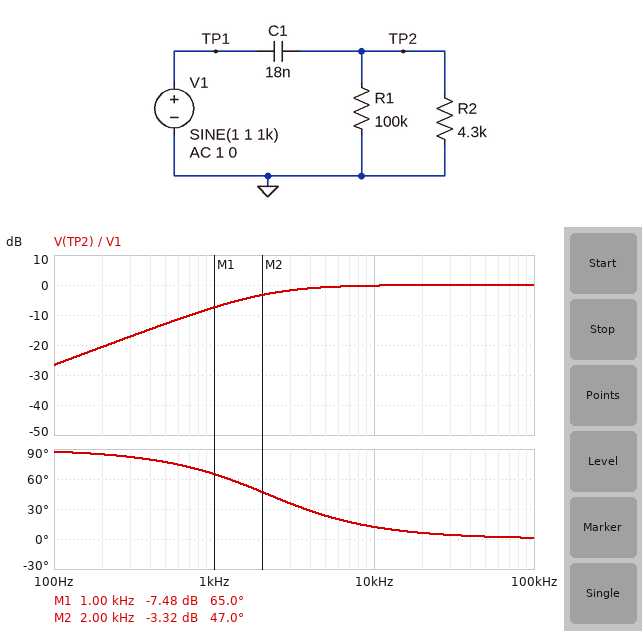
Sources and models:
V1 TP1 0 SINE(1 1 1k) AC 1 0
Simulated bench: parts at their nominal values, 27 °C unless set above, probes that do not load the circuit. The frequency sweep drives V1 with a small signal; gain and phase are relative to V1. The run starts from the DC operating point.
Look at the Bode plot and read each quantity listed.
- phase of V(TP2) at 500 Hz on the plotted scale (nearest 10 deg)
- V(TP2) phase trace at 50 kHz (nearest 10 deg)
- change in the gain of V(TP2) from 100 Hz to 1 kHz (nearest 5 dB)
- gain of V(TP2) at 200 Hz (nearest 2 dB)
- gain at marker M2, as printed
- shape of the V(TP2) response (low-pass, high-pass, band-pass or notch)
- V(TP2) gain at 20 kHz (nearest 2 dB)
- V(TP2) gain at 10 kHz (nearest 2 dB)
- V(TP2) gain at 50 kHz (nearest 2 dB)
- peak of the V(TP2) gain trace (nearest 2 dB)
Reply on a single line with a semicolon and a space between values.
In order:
80 deg; 0 deg; 20 dB; -20 dB; -3.32 dB; high-pass; 0 dB; 0 dB; 0 dB; 0 dB
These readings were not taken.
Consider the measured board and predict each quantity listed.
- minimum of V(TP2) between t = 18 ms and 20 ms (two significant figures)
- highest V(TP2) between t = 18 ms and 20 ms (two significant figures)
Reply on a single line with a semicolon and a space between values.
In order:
-420 mV; 420 mV
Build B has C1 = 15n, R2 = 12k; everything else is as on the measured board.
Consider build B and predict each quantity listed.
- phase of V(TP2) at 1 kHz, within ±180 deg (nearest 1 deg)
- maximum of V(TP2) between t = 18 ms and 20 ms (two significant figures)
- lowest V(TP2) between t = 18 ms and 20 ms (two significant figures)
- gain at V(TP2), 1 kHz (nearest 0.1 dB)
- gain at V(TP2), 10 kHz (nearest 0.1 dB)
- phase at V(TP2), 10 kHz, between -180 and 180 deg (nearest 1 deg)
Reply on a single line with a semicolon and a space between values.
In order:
45 deg; 710 mV; -710 mV; -3.0 dB; 0 dB; 6 deg
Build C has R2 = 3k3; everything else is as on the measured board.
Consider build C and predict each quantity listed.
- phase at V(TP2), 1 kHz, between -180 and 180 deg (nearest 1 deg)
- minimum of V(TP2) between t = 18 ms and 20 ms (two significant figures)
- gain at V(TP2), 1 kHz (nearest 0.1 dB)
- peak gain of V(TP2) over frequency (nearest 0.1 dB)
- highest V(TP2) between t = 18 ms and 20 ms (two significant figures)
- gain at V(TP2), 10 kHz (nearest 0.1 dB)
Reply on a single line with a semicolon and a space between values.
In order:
70 deg; -340 mV; -9.4 dB; 0 dB; 340 mV; -0.3 dB
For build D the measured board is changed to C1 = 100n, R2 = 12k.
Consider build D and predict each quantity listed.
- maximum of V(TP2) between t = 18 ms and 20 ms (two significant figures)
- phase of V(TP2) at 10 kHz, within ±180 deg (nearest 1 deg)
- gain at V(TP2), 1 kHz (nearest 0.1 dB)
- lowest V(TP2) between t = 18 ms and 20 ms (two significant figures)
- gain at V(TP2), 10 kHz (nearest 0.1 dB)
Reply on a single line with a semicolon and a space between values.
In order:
990 mV; 1 deg; -0.1 dB; -990 mV; 0 dB
